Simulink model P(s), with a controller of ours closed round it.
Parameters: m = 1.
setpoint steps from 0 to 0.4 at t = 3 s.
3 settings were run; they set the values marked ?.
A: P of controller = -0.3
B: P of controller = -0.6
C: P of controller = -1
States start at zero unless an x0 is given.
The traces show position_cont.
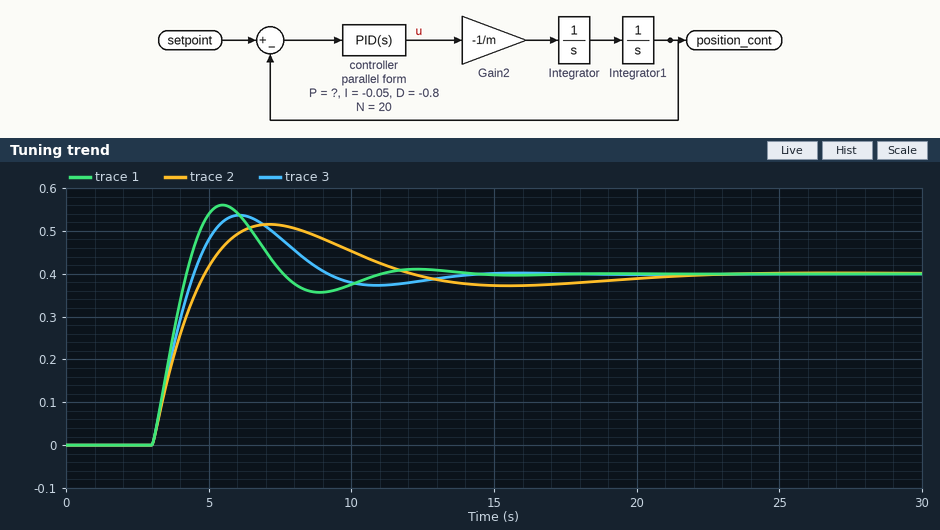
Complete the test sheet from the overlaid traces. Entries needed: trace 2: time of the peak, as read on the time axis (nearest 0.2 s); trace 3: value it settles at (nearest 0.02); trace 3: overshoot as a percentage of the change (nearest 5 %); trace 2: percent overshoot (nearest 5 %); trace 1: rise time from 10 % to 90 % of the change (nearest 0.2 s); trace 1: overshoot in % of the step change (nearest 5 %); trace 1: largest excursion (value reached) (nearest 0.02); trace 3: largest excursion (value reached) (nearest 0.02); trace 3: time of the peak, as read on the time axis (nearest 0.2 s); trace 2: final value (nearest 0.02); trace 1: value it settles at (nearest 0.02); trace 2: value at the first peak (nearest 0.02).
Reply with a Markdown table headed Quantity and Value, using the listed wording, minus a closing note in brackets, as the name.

| Quantity | Value |
|---|---|
| trace 2: time of the peak, as read on the time axis | 7.2 s |
| trace 3: value it settles at | 0.40 |
| trace 3: overshoot as a percentage of the change | 35 % |
| trace 2: percent overshoot | 30 % |
| trace 1: rise time from 10 % to 90 % of the change | 1.0 s |
| trace 1: overshoot in % of the step change | 40 % |
| trace 1: largest excursion (value reached) | 0.56 |
| trace 3: largest excursion (value reached) | 0.54 |
| trace 3: time of the peak, as read on the time axis | 6.0 s |
| trace 2: final value | 0.40 |
| trace 1: value it settles at | 0.40 |
| trace 2: value at the first peak | 0.52 |
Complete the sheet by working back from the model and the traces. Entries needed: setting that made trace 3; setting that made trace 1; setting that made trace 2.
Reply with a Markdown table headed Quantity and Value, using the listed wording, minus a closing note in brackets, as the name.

| Quantity | Value |
|---|---|
| setting that made trace 3 | B |
| setting that made trace 1 | C |
| setting that made trace 2 | A |
